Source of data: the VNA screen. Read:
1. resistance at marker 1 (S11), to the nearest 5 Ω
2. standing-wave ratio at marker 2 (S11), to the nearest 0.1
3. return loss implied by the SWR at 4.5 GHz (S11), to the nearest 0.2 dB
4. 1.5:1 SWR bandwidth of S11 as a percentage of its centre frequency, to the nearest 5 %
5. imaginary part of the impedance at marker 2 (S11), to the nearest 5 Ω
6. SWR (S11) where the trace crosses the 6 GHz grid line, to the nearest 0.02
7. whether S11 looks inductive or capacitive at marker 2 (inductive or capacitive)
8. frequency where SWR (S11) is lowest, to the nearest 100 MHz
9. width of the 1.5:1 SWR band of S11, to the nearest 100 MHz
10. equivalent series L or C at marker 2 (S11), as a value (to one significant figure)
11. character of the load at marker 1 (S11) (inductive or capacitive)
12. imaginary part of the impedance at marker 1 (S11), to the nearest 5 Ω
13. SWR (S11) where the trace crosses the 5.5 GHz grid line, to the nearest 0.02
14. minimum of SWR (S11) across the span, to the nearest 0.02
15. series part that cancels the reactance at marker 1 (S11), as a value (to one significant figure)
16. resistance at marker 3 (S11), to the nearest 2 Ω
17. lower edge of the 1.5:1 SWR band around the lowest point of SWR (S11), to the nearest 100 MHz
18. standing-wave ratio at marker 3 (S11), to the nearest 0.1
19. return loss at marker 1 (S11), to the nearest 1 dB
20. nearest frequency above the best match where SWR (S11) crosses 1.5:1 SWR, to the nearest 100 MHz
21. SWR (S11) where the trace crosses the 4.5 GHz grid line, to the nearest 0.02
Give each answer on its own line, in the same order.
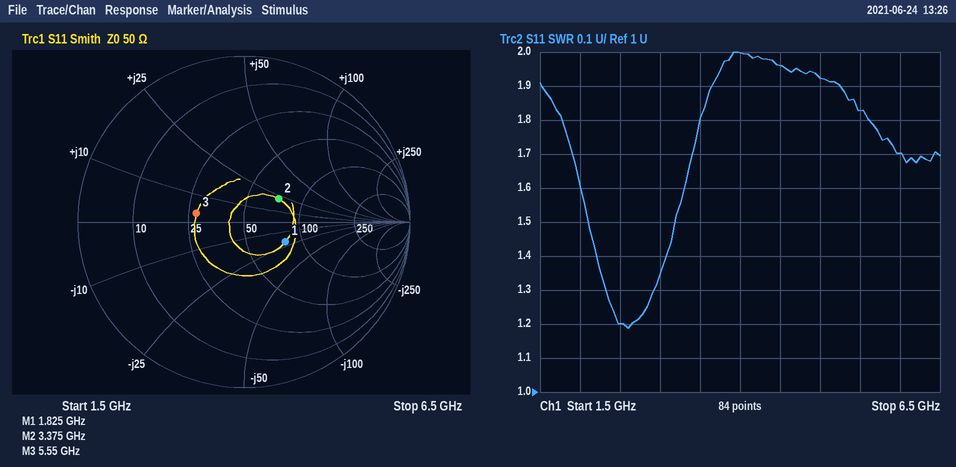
80 Ω
1.7
9.8 dB
40 %
+20 Ω
1.70
inductive
2.6 GHz
1.1 GHz
1 nH
capacitive
-20 Ω
1.82
1.18
2 nH
28 Ω
2.1 GHz
1.8
11 dB
3.2 GHz
1.96
